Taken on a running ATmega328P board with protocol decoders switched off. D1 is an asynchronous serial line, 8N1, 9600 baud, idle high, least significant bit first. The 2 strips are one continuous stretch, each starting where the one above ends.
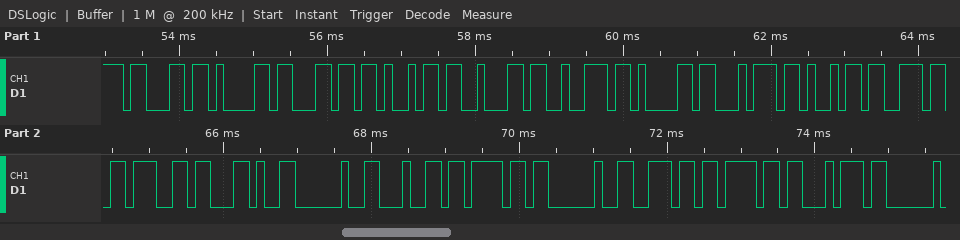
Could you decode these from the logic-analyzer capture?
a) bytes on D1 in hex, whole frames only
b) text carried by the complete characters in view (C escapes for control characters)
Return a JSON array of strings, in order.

["63 61 6C 69 62 72 61 74 69 6E 67 2C 20 64 6F 20 6E 6F 74", "\"calibrating, do not\""]
